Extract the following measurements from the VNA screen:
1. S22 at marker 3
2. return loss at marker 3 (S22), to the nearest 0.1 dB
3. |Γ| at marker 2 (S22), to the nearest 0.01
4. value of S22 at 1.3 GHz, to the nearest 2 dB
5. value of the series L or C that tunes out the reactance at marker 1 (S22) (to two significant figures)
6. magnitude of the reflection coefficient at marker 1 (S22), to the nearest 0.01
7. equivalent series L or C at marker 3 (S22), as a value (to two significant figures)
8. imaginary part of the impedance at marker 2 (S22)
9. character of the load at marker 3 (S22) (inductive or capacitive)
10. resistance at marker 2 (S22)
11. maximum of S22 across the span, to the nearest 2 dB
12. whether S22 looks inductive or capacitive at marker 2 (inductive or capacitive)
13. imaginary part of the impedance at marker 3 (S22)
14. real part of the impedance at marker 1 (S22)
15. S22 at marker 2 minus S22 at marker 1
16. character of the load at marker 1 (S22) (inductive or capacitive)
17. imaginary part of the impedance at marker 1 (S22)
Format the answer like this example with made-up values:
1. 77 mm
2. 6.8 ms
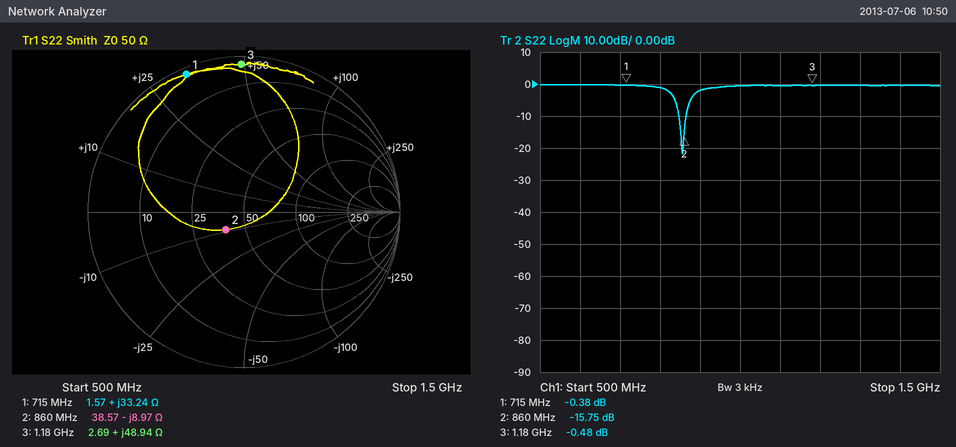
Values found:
1. -0.48 dB
2. 0.5 dB
3. 0.16
4. 0 dB
5. 6.7 pF
6. 0.96
7. 6.6 nH
8. -8.97 Ω
9. inductive
10. 38.57 Ω
11. 0 dB
12. capacitive
13. +48.94 Ω
14. 1.57 Ω
15. -15.37 dB
16. inductive
17. +33.24 Ω
